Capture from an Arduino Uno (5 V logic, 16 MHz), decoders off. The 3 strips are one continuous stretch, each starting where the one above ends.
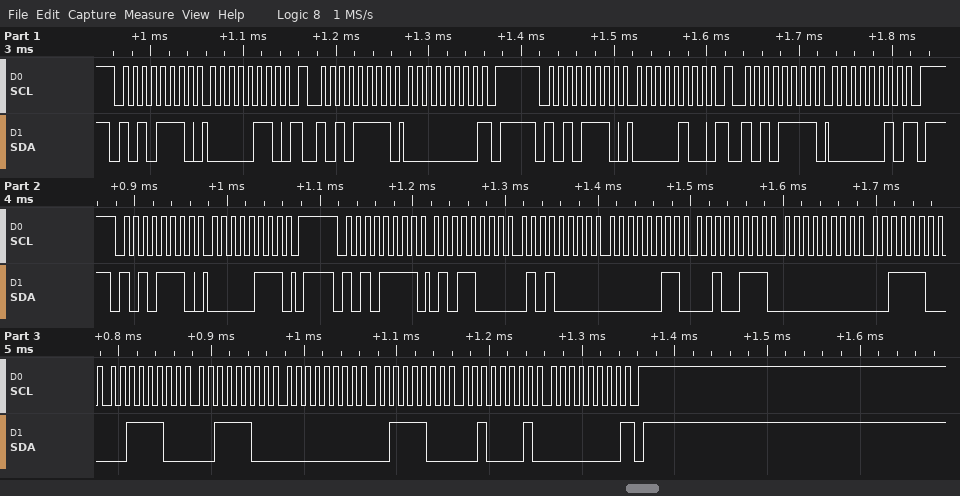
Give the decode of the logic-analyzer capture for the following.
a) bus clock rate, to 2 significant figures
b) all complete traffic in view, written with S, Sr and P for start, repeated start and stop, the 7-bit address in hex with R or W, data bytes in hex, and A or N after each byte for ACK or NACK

100 kHz
S 57W A 06 A Sr 57R A 00 N P S 57W A 04 A Sr 57R A 02 N P S 57W A 07 A P S 57R A 58 A 50 A 03 A 27 A 00 A 3C A 3C A 3C A 00 A 3C A 21 A 00 N P
